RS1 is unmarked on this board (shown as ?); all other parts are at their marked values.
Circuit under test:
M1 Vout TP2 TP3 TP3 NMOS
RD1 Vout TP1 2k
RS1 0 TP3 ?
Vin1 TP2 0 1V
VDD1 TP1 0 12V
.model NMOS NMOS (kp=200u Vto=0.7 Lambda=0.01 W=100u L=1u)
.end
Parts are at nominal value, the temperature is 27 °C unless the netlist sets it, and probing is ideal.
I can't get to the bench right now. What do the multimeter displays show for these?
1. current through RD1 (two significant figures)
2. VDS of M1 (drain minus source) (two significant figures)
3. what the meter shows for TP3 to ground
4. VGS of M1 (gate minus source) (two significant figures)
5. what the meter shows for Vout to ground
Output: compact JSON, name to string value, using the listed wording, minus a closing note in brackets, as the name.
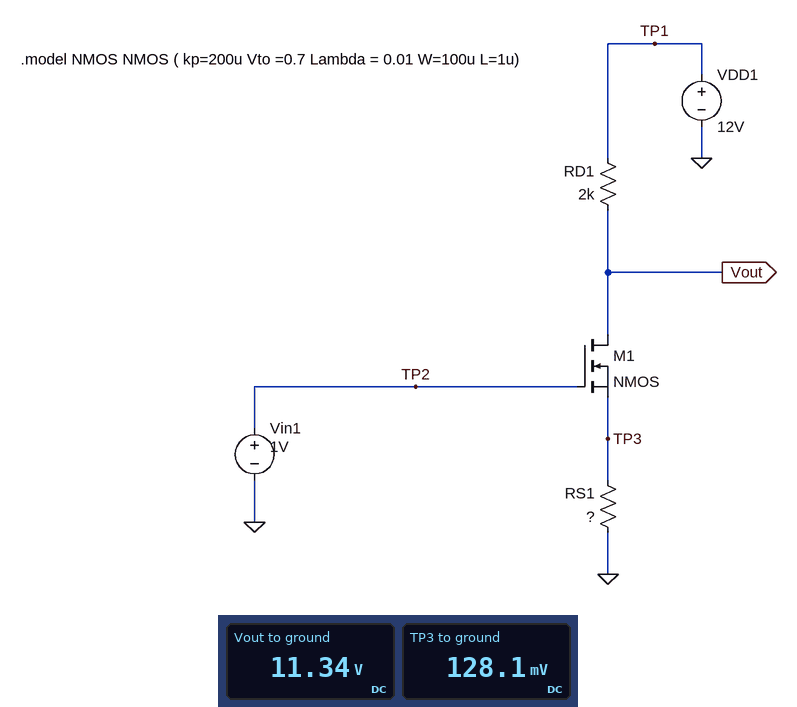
{"current through RD1": "330 µA", "VDS of M1 (drain minus source)": "11 V", "what the meter shows for TP3 to ground": "128.1 mV", "VGS of M1 (gate minus source)": "870 mV", "what the meter shows for Vout to ground": "11.34 V"}
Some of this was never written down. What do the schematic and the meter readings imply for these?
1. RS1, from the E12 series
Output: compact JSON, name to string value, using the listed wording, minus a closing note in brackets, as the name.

{"RS1, from the E12 series": "390 Ω"}
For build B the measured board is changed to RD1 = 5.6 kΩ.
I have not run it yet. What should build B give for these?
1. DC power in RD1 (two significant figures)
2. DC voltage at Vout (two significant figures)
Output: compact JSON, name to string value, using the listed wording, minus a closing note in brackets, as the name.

{"DC power in RD1": "600 µW", "DC voltage at Vout": "10 V"}
